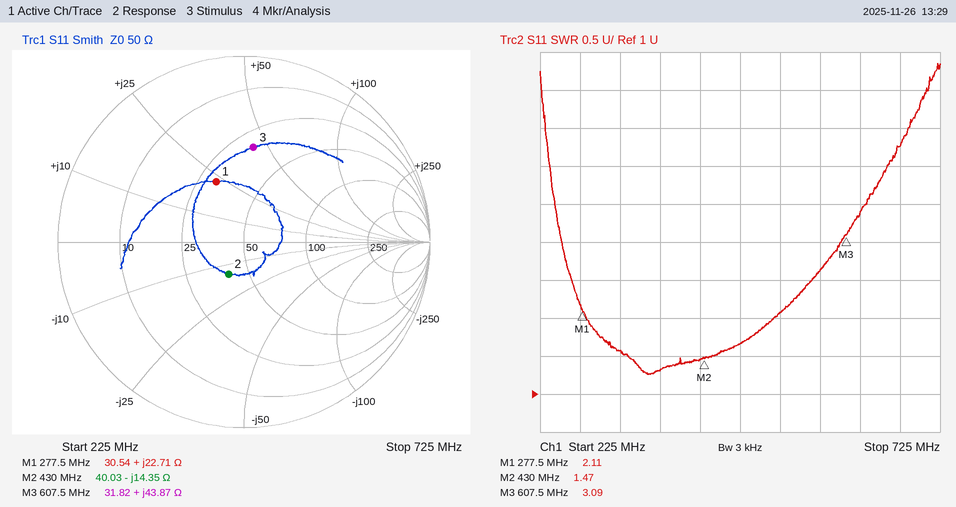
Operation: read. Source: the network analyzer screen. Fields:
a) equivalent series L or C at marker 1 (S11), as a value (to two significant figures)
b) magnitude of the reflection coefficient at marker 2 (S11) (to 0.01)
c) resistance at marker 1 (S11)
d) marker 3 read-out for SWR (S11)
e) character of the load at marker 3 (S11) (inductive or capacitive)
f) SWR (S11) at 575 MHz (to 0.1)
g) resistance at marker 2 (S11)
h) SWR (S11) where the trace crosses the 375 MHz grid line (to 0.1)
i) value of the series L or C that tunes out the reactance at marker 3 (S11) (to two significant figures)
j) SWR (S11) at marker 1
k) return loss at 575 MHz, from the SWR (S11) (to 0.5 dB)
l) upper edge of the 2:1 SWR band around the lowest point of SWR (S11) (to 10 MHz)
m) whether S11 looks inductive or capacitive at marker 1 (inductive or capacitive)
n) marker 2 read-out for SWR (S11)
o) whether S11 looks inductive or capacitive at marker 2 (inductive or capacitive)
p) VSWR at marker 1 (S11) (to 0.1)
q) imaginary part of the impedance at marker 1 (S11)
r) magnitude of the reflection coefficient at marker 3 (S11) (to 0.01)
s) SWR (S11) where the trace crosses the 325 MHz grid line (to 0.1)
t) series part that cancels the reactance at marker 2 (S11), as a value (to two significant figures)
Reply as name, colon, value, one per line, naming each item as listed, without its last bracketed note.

equivalent series L or C at marker 1 (S11), as a value: 13 nH
magnitude of the reflection coefficient at marker 2 (S11): 0.19
resistance at marker 1: 30.54 Ω
marker 3 read-out for SWR: 3.09
character of the load at marker 3 (S11): inductive
SWR (S11) at 575 MHz: 2.6
resistance at marker 2: 40.03 Ω
SWR (S11) where the trace crosses the 375 MHz grid line: 1.3
value of the series L or C that tunes out the reactance at marker 3 (S11): 6.0 pF
SWR (S11) at marker 1: 2.11
return loss at 575 MHz, from the SWR (S11): 7.0 dB
upper edge of the 2:1 SWR band around the lowest point of SWR (S11): 520 MHz
whether S11 looks inductive or capacitive at marker 1: inductive
marker 2 read-out for SWR: 1.47
whether S11 looks inductive or capacitive at marker 2: capacitive
VSWR at marker 1 (S11): 2.1
imaginary part of the impedance at marker 1: +22.71 Ω
magnitude of the reflection coefficient at marker 3 (S11): 0.51
SWR (S11) where the trace crosses the 325 MHz grid line: 1.6
series part that cancels the reactance at marker 2 (S11), as a value: 5.3 nH
